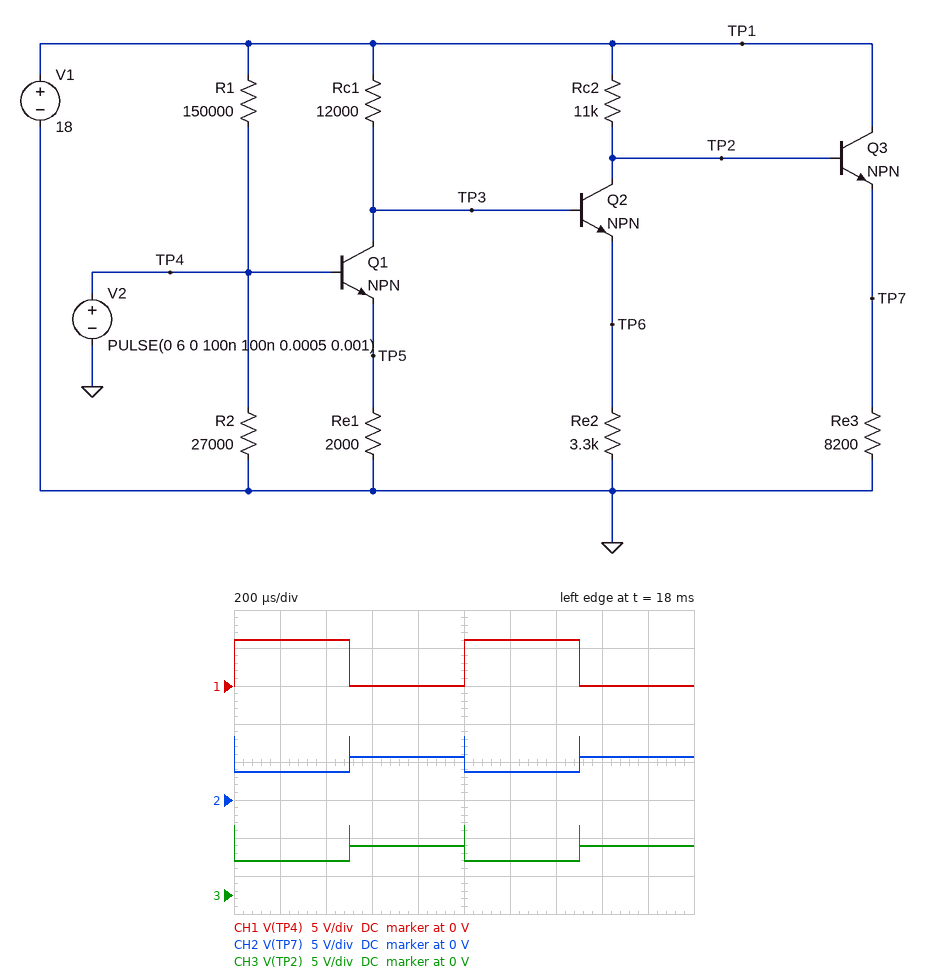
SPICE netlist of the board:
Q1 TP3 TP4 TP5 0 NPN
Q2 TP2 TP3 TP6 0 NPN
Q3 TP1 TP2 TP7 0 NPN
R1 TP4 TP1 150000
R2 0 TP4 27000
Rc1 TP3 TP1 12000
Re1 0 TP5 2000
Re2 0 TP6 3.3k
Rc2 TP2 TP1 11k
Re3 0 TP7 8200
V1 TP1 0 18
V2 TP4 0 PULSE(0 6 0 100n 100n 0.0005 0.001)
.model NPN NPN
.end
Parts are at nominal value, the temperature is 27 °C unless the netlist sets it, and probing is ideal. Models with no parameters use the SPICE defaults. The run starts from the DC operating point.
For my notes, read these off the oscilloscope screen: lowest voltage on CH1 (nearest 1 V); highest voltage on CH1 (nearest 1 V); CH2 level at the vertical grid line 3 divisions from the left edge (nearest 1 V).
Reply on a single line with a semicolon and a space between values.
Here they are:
0 V; 6 V; 6 V
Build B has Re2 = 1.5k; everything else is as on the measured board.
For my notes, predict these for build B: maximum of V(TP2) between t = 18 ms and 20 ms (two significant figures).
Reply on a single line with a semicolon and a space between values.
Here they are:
4.4 V
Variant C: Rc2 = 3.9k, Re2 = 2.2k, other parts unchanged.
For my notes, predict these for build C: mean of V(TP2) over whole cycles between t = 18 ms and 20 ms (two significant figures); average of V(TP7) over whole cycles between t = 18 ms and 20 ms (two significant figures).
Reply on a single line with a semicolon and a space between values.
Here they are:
8.9 V; 8.1 V
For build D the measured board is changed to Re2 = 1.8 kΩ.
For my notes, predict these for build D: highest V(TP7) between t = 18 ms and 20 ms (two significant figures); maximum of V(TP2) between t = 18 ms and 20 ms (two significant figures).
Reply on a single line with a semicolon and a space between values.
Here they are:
3.7 V; 4.4 V
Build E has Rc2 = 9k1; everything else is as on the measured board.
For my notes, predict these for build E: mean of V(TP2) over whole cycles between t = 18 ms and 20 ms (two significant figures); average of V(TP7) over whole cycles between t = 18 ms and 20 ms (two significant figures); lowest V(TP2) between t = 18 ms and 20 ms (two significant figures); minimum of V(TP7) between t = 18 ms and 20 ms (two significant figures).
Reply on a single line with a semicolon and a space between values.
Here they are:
6.4 V; 5.6 V; 5.8 V; 5.1 V
